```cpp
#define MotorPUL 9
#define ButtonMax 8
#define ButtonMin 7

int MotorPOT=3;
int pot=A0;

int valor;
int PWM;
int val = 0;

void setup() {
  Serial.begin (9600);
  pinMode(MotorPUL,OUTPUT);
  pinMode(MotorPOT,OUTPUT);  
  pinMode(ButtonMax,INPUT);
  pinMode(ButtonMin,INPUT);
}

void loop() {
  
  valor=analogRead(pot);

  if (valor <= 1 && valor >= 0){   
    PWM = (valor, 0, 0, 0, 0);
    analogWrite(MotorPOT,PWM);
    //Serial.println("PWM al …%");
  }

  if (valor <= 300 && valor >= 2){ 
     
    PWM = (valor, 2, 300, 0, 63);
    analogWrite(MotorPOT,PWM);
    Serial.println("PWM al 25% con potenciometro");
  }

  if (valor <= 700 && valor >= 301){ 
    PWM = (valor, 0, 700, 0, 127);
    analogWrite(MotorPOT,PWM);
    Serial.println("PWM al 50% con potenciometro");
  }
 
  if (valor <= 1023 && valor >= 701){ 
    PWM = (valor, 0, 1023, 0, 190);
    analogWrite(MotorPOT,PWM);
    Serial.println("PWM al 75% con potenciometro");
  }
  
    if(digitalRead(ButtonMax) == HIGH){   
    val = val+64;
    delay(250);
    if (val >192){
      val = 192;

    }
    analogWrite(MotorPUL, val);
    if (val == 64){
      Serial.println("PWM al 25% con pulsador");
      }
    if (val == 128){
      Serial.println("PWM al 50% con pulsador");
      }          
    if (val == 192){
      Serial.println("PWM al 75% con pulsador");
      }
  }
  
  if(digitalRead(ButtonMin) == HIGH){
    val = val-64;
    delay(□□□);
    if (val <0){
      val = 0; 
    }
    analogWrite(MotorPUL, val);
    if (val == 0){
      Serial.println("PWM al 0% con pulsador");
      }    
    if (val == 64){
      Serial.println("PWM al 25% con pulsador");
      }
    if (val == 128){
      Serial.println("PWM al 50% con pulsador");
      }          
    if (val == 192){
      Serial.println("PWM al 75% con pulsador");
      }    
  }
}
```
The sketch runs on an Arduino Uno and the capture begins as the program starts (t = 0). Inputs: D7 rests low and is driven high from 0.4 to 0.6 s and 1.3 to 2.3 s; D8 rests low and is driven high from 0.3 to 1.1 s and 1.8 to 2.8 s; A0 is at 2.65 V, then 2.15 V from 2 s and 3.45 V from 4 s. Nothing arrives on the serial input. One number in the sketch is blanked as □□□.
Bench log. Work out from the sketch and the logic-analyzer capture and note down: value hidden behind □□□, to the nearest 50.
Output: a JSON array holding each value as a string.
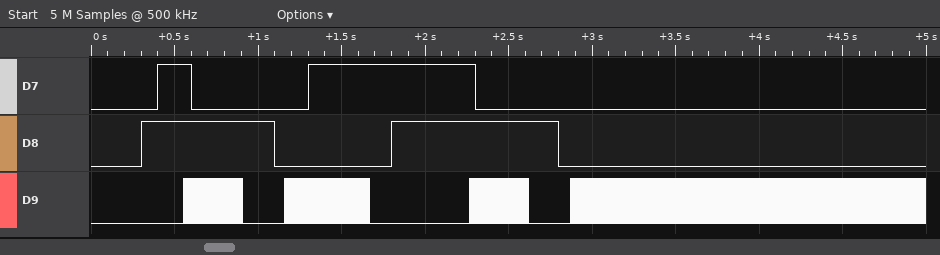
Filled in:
["350"]
